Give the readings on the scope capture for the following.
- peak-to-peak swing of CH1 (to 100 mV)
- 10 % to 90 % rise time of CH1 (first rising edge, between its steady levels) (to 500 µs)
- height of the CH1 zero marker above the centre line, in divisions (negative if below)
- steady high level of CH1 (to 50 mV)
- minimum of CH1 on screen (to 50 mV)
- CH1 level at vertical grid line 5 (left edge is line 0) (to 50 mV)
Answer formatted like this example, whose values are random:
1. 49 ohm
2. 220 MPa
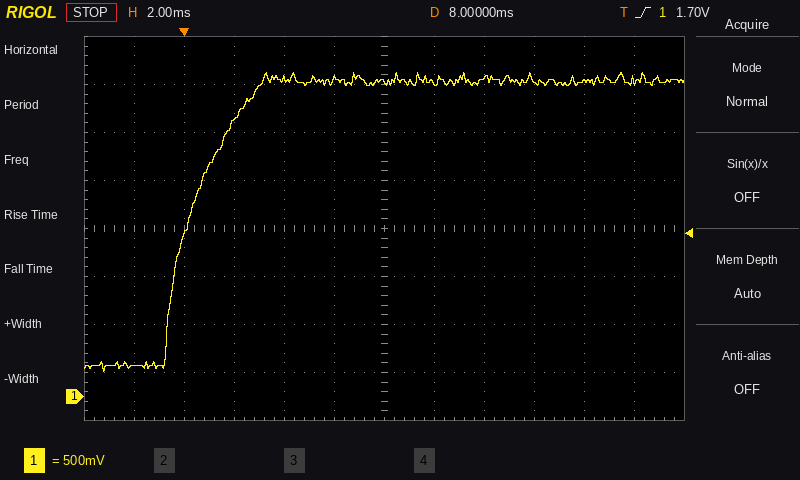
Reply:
1. 3.10 V
2. 3.0 ms
3. -3.5 div
4. 3.30 V
5. 250 mV
6. 3.30 V
